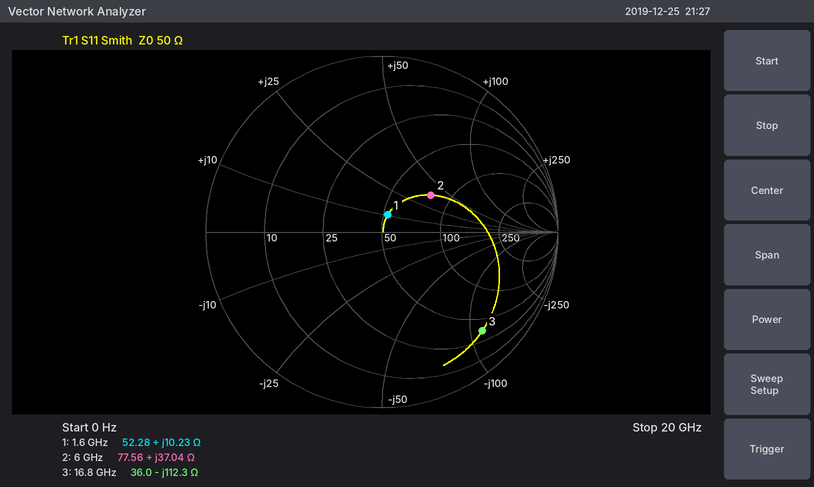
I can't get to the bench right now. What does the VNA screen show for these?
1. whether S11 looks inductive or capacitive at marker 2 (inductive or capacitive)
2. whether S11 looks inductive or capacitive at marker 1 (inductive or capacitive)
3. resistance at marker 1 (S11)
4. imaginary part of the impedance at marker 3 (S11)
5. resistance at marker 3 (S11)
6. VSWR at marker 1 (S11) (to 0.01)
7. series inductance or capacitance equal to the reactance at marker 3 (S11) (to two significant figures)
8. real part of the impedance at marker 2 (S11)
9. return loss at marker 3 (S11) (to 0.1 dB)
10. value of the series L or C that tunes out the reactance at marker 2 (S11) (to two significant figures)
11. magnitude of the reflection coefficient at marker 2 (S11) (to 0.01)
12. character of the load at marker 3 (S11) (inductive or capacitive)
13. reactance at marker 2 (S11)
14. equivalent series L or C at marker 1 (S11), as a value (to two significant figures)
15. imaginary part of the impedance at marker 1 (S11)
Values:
inductive
inductive
52.28 Ω
-112.3 Ω
36.0 Ω
1.23
84 fF
77.56 Ω
1.9 dB
720 fF
0.35
capacitive
+37.04 Ω
1.0 nH
+10.23 Ω
